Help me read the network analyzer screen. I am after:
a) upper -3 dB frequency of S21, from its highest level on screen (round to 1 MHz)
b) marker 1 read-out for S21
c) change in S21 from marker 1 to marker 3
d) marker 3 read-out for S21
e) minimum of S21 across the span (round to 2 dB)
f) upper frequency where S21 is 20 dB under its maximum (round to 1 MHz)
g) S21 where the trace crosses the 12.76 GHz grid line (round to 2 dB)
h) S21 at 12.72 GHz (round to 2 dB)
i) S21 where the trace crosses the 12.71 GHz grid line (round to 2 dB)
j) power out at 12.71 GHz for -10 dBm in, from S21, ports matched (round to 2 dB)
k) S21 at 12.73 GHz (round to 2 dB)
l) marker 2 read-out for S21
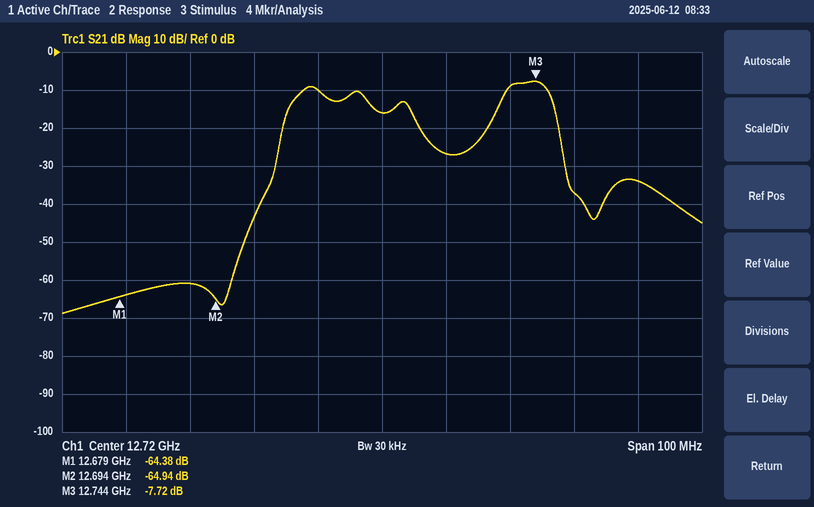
12.746 GHz
-64.38 dB
56.66 dB
-7.72 dB
-68 dB
12.748 GHz
-34 dB
-16 dB
-10 dB
-20 dBm
-26 dB
-64.94 dB
